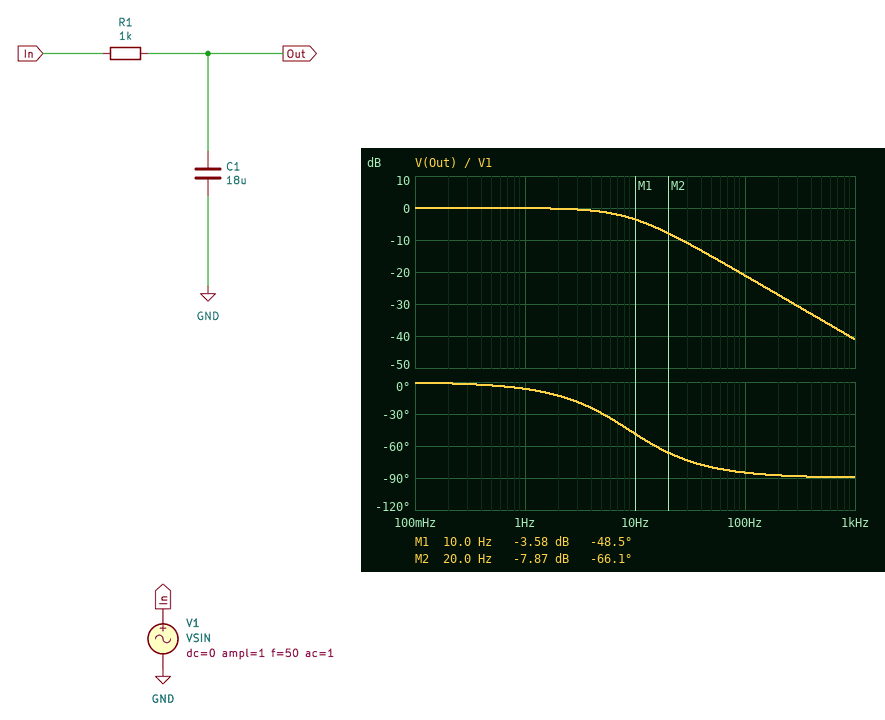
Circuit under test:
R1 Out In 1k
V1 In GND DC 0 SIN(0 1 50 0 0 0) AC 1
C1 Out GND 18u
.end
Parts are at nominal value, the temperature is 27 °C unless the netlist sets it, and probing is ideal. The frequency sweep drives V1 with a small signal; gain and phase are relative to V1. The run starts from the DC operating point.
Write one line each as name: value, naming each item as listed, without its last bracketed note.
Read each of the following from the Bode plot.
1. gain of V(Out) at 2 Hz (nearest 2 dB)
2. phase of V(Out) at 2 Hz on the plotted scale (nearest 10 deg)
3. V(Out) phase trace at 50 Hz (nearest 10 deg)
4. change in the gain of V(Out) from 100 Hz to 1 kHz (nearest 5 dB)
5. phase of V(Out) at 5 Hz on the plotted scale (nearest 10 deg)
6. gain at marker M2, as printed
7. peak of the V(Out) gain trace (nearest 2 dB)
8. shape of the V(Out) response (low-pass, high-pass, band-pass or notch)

gain of V(Out) at 2 Hz: 0 dB
phase of V(Out) at 2 Hz on the plotted scale: -10 deg
V(Out) phase trace at 50 Hz: -80 deg
change in the gain of V(Out) from 100 Hz to 1 kHz: -20 dB
phase of V(Out) at 5 Hz on the plotted scale: -30 deg
gain at marker M2, as printed: -7.87 dB
peak of the V(Out) gain trace: 0 dB
shape of the V(Out) response: low-pass
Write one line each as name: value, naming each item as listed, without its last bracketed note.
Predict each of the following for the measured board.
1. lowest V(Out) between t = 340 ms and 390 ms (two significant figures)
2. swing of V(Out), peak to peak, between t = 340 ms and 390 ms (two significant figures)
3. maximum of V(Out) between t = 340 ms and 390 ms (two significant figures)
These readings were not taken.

lowest V(Out) between t = 340 ms and 390 ms: -170 mV
swing of V(Out), peak to peak, between t = 340 ms and 390 ms: 350 mV
maximum of V(Out) between t = 340 ms and 390 ms: 170 mV
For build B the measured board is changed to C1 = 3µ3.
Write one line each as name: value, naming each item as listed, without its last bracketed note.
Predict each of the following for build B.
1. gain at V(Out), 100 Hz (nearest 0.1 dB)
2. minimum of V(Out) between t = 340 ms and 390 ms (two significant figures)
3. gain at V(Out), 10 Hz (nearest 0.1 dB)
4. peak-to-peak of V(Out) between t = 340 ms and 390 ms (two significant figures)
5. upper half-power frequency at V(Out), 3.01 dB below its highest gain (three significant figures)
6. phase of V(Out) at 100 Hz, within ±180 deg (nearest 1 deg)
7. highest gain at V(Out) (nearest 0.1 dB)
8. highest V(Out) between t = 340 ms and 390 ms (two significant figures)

gain at V(Out), 100 Hz: -7.2 dB
minimum of V(Out) between t = 340 ms and 390 ms: -690 mV
gain at V(Out), 10 Hz: -0.2 dB
peak-to-peak of V(Out) between t = 340 ms and 390 ms: 1.4 V
upper half-power frequency at V(Out), 3.01 dB below its highest gain: 48.2 Hz
phase of V(Out) at 100 Hz, within ±180 deg: -64 deg
highest gain at V(Out): 0 dB
highest V(Out) between t = 340 ms and 390 ms: 690 mV
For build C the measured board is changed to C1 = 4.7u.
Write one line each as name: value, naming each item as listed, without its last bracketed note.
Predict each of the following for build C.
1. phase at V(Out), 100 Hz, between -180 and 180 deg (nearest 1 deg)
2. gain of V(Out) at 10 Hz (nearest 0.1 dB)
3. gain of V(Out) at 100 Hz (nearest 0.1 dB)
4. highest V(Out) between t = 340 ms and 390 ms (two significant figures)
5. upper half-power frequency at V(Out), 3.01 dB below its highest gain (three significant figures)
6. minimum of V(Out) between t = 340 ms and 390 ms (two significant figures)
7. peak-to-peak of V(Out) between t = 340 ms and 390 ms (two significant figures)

phase at V(Out), 100 Hz, between -180 and 180 deg: -71 deg
gain of V(Out) at 10 Hz: -0.4 dB
gain of V(Out) at 100 Hz: -9.9 dB
highest V(Out) between t = 340 ms and 390 ms: 560 mV
upper half-power frequency at V(Out), 3.01 dB below its highest gain: 33.9 Hz
minimum of V(Out) between t = 340 ms and 390 ms: -560 mV
peak-to-peak of V(Out) between t = 340 ms and 390 ms: 1.1 V
